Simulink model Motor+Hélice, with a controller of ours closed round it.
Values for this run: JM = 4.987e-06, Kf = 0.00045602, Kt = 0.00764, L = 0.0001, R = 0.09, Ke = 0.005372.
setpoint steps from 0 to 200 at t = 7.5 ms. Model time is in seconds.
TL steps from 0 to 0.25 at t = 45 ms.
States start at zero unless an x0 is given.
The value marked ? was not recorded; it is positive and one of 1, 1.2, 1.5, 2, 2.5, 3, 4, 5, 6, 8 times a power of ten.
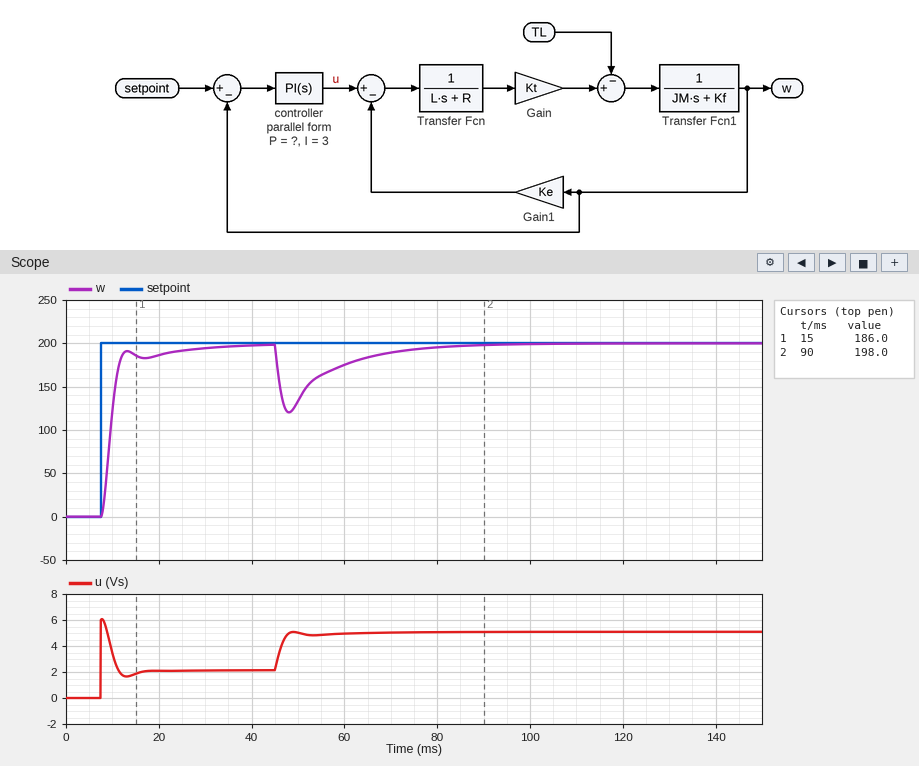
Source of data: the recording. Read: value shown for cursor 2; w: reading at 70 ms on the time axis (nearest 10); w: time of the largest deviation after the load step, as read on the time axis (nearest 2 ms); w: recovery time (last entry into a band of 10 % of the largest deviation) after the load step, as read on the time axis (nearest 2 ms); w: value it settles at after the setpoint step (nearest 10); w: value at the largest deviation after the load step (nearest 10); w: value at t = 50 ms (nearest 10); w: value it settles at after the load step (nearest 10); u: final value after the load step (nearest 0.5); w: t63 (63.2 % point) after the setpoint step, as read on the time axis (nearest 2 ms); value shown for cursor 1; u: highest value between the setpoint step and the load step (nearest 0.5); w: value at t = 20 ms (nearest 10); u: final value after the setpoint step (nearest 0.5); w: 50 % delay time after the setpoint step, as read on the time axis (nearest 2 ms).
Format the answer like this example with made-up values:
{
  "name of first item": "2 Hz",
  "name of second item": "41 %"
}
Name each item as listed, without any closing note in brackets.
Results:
{
  "value shown for cursor 2": "198.0",
  "w: reading at 70 ms on the time axis": "190",
  "w: time of the largest deviation after the load step, as read on the time axis": "48 ms",
  "w: recovery time (last entry into a band of 10 % of the largest deviation) after the load step, as read on the time axis": "74 ms",
  "w: value it settles at after the setpoint step": "200",
  "w: value at the largest deviation after the load step": "120",
  "w: value at t = 50 ms": "130",
  "w: value it settles at after the load step": "200",
  "u: final value after the load step": "5.0",
  "w: t63 (63.2 % point) after the setpoint step, as read on the time axis": "10 ms",
  "value shown for cursor 1": "186.0",
  "u: highest value between the setpoint step and the load step": "6.0",
  "w: value at t = 20 ms": "190",
  "u: final value after the setpoint step": "2.0",
  "w: 50 % delay time after the setpoint step, as read on the time axis": "10 ms"
}
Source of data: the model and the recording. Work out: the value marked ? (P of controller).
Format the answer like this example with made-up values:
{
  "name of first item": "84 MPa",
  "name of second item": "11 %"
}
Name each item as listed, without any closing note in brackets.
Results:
{
  "the value marked ?": "0.03"
}
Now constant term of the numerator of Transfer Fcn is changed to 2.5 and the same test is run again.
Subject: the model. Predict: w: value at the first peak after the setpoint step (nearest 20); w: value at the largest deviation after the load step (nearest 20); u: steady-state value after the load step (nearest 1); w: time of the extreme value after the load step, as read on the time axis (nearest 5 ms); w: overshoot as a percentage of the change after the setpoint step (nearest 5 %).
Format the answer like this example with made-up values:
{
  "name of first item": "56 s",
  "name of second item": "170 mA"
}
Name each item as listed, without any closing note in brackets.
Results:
{
  "w: value at the first peak after the setpoint step": "220",
  "w: value at the largest deviation after the load step": "160",
  "u: steady-state value after the load step": "3",
  "w: time of the extreme value after the load step, as read on the time axis": "45 ms",
  "w: overshoot as a percentage of the change after the setpoint step": "10 %"
}
